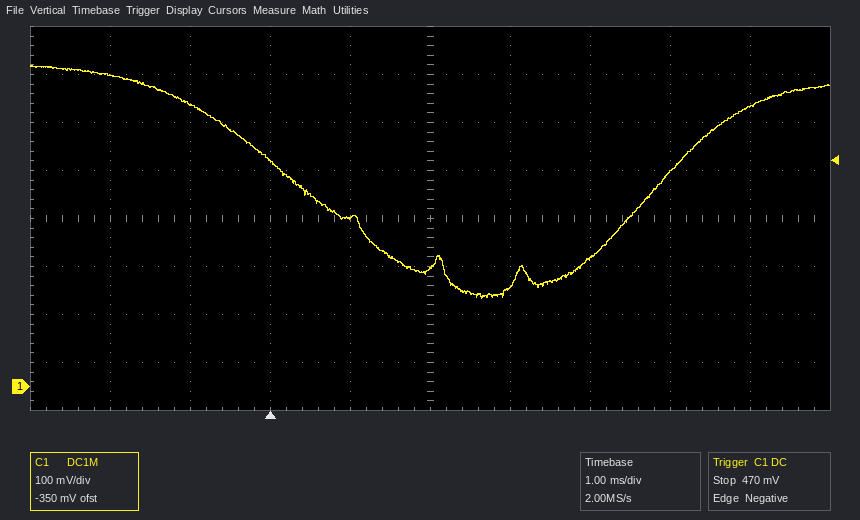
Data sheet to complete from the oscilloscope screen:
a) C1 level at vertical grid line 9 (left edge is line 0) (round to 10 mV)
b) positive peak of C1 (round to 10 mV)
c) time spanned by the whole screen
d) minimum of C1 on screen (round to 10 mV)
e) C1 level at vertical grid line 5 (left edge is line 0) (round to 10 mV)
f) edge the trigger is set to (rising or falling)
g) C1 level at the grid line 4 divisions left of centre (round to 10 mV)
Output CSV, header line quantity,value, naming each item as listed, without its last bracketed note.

quantity,value
C1 level at vertical grid line 9 (left edge is line 0),580 mV
positive peak of C1,670 mV
time spanned by the whole screen,10 ms
minimum of C1 on screen,180 mV
C1 level at vertical grid line 5 (left edge is line 0),250 mV
edge the trigger is set to,falling
C1 level at the grid line 4 divisions left of centre,650 mV
